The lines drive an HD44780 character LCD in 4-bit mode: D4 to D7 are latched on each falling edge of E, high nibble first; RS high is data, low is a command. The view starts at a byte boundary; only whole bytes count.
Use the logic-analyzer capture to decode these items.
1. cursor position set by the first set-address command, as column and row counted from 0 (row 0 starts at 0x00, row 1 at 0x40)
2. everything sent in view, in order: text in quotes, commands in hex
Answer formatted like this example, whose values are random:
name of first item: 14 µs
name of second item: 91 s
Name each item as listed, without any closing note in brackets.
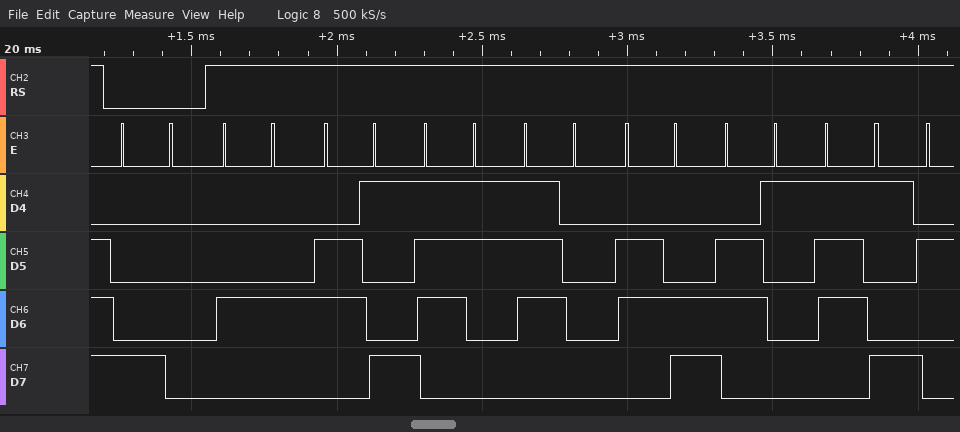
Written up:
cursor position set by the first set-address command, as column and row counted from 0: column 0, row 0
everything sent in view, in order: text in quotes, commands in hex: 0x80 "Display"
